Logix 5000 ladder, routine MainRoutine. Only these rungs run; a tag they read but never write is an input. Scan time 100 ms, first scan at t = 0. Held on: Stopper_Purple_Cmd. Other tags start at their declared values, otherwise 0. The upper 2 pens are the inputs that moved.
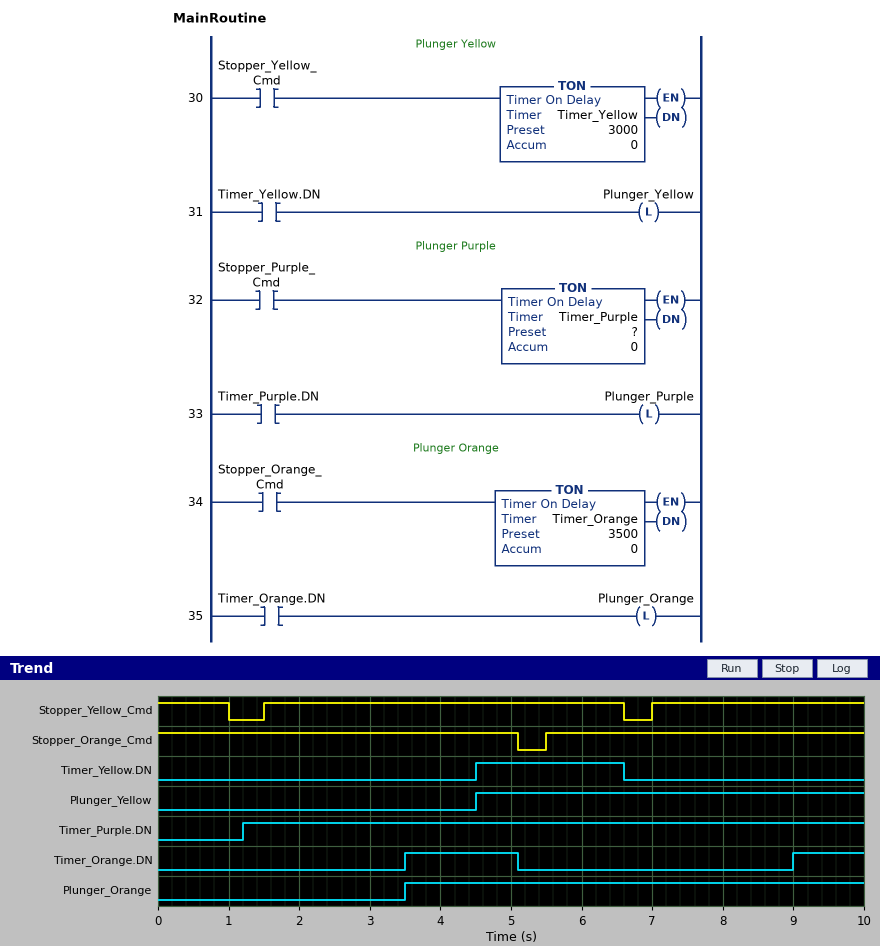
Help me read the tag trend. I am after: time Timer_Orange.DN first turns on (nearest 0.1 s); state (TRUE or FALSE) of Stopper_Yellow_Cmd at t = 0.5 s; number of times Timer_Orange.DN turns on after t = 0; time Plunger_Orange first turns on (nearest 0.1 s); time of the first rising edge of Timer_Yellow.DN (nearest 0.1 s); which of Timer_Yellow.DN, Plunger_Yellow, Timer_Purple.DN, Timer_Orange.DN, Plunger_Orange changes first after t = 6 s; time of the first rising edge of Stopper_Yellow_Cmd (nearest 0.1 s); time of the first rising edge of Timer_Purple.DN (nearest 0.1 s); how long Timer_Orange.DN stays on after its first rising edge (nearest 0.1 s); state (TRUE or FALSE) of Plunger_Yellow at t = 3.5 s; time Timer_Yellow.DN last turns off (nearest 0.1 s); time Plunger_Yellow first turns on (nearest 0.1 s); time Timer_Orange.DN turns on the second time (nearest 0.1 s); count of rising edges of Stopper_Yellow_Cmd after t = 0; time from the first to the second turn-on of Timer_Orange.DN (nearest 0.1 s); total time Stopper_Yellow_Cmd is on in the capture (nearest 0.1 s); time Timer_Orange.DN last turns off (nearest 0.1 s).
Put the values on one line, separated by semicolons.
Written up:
3.5 s; TRUE; 2; 3.5 s; 4.5 s; Timer_Yellow.DN; 1.5 s; 1.2 s; 1.6 s; FALSE; 6.6 s; 4.5 s; 9.0 s; 2; 5.5 s; 9.1 s; 5.1 s
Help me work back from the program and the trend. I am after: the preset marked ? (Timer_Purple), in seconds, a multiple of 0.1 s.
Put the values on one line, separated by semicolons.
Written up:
1.2 s
